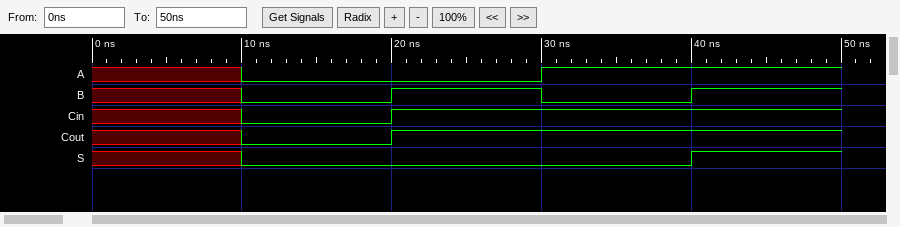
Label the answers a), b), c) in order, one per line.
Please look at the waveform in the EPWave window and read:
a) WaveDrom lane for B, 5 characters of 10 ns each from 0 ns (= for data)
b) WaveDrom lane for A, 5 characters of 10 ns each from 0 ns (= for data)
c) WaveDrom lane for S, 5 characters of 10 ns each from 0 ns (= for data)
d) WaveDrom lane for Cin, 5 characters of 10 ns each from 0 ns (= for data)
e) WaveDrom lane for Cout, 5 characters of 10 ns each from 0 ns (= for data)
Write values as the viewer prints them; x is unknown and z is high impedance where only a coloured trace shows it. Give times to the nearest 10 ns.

a) {name: 'B', wave: 'x0101'}
b) {name: 'A', wave: 'x0.1.'}
c) {name: 'S', wave: 'x0..1'}
d) {name: 'Cin', wave: 'x01..'}
e) {name: 'Cout', wave: 'x01..'}
